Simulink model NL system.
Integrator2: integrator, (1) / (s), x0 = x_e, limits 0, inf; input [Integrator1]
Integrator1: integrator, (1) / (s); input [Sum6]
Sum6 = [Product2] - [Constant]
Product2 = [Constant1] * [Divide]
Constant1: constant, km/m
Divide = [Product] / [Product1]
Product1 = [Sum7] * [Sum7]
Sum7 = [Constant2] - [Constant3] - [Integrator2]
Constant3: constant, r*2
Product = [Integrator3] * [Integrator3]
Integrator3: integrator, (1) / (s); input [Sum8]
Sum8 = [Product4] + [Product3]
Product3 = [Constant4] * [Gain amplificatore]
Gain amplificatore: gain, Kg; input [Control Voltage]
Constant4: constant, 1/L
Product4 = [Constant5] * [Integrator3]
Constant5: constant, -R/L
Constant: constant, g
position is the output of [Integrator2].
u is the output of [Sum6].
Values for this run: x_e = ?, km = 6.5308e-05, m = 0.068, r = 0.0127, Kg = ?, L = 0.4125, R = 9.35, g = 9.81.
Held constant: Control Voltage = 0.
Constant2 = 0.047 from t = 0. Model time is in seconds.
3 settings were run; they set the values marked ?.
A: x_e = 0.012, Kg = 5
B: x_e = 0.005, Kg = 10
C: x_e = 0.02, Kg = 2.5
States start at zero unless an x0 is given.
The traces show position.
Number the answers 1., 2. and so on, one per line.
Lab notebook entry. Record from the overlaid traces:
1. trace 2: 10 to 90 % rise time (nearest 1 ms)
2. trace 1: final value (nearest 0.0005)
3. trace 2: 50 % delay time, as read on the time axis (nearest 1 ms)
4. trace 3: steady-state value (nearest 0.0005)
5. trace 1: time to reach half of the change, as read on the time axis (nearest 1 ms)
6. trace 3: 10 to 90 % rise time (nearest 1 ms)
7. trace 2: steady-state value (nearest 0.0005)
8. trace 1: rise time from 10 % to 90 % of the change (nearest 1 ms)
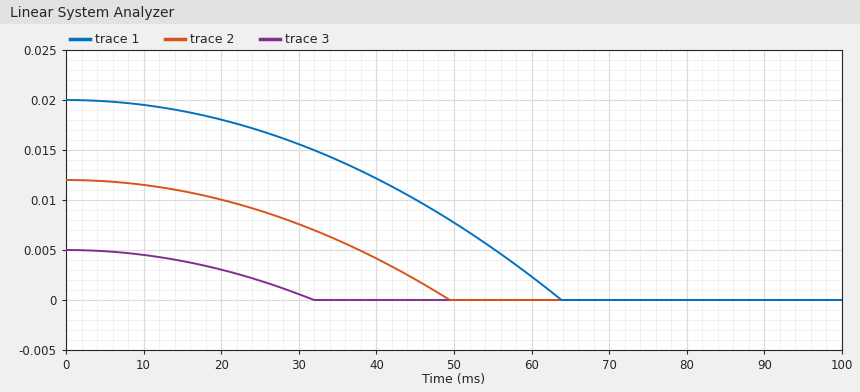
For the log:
1. 31 ms
2. 0.0000
3. 35 ms
4. 0.0000
5. 45 ms
6. 20 ms
7. 0.0000
8. 40 ms
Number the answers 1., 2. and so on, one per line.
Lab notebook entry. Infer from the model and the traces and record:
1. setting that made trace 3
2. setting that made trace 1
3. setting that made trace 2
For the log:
1. B
2. C
3. A
